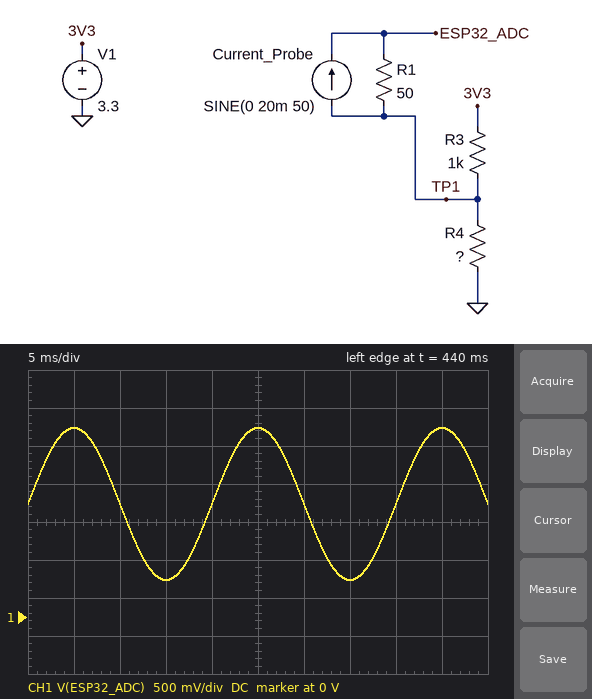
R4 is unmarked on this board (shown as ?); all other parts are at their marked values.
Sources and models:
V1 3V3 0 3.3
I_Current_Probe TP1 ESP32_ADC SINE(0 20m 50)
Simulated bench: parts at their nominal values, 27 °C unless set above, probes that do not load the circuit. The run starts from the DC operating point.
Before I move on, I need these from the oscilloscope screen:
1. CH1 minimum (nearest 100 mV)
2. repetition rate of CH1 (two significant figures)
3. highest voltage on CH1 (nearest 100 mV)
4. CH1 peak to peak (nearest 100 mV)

500 mV
50 Hz
2.5 V
2.0 V
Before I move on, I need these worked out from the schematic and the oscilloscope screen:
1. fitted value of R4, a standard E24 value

820 Ω
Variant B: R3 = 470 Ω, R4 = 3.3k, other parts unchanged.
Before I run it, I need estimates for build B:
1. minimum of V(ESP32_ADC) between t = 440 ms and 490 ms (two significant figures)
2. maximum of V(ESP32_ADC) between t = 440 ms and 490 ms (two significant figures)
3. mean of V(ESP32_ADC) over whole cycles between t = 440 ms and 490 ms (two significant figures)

1.9 V
3.9 V
2.9 V
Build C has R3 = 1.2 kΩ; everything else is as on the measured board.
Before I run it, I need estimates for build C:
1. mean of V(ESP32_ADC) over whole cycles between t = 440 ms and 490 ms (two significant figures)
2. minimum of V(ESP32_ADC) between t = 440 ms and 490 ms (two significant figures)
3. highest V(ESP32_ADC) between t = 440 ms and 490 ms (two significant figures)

1.3 V
340 mV
2.3 V
